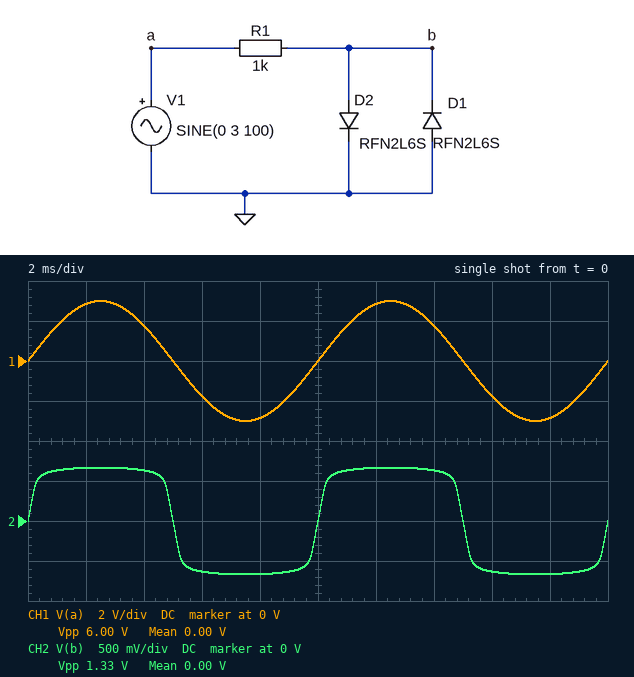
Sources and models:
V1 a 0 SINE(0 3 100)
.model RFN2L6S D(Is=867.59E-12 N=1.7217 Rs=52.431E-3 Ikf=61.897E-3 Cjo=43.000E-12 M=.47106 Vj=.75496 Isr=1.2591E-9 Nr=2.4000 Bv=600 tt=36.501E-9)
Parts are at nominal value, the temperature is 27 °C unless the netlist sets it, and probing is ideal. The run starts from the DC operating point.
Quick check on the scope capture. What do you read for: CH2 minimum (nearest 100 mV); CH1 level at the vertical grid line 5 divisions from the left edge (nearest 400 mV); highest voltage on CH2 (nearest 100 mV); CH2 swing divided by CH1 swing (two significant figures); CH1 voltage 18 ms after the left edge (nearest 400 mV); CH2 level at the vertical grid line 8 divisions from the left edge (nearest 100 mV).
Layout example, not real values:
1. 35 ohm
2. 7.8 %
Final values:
1. -700 mV
2. 0 V
3. 700 mV
4. 0.22
5. -2.8 V
6. -600 mV
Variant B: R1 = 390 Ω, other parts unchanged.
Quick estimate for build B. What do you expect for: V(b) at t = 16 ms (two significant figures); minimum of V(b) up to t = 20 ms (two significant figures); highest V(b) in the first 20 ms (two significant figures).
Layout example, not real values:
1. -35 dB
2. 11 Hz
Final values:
1. -680 mV
2. -710 mV
3. 710 mV
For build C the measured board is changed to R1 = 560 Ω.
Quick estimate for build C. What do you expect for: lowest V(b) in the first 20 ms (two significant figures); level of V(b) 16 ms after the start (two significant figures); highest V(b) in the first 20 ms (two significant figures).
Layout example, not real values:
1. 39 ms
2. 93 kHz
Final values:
1. -700 mV
2. -660 mV
3. 700 mV
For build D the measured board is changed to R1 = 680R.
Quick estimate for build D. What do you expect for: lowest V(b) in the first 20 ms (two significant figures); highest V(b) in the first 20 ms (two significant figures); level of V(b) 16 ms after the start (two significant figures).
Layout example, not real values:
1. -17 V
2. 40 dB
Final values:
1. -690 mV
2. 690 mV
3. -650 mV
